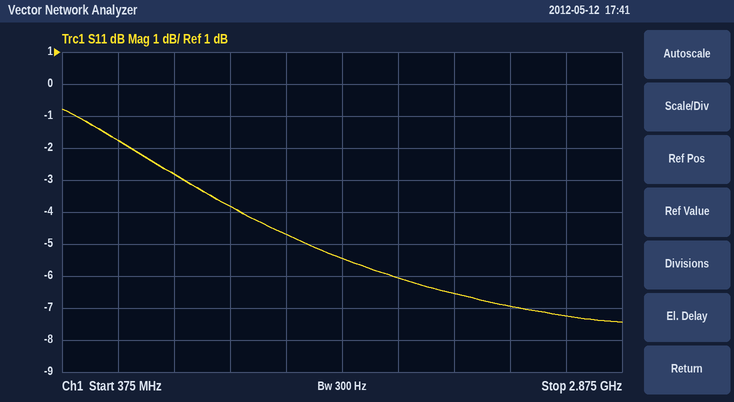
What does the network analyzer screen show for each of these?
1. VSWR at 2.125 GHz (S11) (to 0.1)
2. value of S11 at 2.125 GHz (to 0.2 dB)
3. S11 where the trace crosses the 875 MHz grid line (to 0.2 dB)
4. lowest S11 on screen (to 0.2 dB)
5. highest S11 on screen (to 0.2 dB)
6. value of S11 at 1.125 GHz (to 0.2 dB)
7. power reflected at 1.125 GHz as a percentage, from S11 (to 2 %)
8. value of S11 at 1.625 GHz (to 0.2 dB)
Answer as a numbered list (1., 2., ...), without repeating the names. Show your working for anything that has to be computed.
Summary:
1. |Γ| = 10^(-6.6/20) = 0.4677; VSWR = (1 + 0.4677)/(1 − 0.4677) ≈ 2.8
2. -6.6 dB
3. -2.8 dB
4. -7.4 dB
5. -0.8 dB
6. -3.8 dB
7. 10^(-3.8/10) ≈ 42 %
8. -5.4 dB
